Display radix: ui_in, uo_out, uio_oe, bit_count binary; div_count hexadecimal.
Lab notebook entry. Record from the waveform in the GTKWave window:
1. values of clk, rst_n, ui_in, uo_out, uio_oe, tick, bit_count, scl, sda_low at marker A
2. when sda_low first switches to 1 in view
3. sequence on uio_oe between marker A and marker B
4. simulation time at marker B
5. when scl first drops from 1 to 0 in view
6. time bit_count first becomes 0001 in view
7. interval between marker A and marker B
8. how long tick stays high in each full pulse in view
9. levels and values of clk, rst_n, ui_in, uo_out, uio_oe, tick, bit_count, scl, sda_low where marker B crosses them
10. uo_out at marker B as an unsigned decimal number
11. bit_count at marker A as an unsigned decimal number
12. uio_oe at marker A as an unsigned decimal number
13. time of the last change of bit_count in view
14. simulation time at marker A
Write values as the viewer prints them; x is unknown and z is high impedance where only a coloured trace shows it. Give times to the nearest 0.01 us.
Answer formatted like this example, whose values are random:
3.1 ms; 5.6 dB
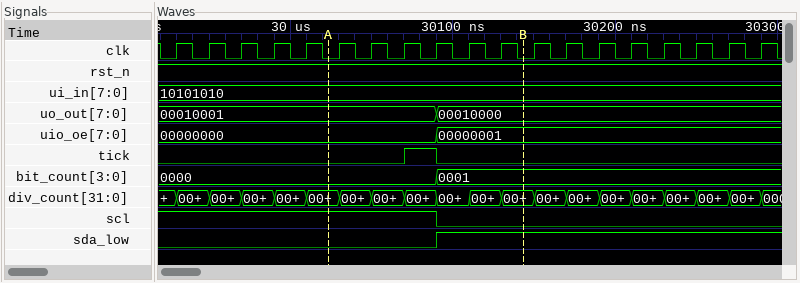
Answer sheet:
clk=0, rst_n=1, ui_in=10101010, uo_out=00010001, uio_oe=00000000, tick=0, bit_count=0000, scl=1, sda_low=0; 30.09 us; 00000000, 00000001; 30.14 us; 30.09 us; 30.09 us; 0.12 us; 0.02 us; clk=0, rst_n=1, ui_in=10101010, uo_out=00010000, uio_oe=00000001, tick=0, bit_count=0001, scl=0, sda_low=1; 16; 0; 0; 30.09 us; 30.02 us
